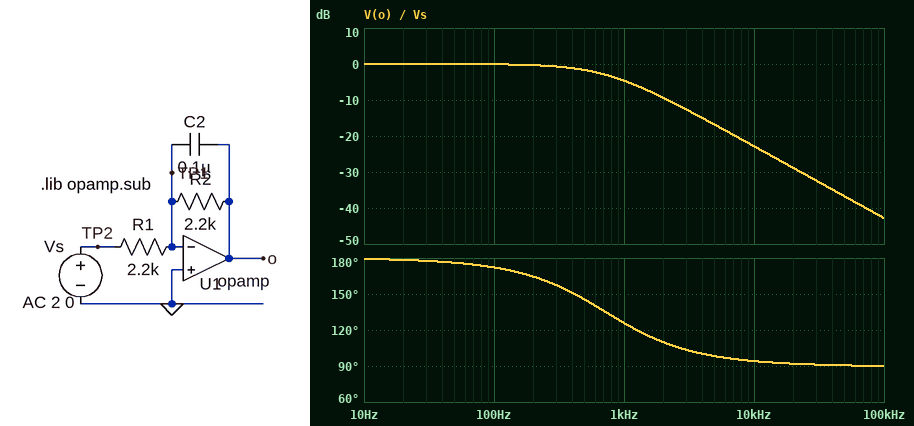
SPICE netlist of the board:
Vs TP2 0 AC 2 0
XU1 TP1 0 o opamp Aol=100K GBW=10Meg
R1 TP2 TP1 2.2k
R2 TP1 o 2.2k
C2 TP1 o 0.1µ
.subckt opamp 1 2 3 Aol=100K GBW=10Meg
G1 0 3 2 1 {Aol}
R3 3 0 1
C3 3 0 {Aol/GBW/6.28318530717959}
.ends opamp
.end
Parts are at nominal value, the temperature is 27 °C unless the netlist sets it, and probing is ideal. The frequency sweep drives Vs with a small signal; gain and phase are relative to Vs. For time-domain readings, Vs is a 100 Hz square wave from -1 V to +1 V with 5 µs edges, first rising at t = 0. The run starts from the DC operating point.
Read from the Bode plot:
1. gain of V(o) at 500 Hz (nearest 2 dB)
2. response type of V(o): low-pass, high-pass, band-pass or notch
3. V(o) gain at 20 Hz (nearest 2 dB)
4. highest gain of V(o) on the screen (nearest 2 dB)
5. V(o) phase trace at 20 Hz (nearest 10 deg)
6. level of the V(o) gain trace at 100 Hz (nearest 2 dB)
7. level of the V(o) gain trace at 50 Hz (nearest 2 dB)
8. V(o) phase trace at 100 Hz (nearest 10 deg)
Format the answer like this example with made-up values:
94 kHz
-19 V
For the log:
-2 dB
low-pass
0 dB
0 dB
180 deg
0 dB
0 dB
170 deg
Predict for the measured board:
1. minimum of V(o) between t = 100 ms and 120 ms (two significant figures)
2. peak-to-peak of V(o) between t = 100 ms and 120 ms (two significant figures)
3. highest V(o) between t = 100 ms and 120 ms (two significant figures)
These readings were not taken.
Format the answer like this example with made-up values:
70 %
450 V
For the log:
-1.0 V
2.0 V
1.0 V
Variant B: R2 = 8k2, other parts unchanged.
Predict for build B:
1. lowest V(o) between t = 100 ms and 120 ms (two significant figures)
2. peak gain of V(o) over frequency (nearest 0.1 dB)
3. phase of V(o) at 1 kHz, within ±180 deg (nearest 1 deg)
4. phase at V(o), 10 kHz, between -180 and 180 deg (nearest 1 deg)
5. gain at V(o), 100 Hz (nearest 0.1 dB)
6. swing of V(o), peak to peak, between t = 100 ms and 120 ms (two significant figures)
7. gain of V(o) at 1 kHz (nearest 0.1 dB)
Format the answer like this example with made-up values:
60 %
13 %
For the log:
-3.7 V
11.4 dB
101 deg
91 deg
10.4 dB
7.4 V
-3.0 dB
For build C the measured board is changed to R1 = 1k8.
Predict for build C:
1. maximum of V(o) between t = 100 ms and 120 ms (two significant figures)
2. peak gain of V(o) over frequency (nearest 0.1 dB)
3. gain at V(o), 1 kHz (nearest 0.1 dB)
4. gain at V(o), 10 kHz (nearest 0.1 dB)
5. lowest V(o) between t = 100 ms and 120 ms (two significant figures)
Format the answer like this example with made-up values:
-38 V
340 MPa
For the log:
1.2 V
1.7 dB
-2.9 dB
-21.1 dB
-1.2 V
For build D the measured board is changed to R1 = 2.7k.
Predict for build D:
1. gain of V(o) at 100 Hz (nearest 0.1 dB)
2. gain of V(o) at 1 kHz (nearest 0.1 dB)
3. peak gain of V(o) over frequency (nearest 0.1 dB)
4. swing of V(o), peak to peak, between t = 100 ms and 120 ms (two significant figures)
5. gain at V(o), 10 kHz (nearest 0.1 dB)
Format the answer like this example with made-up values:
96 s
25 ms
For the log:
-1.9 dB
-6.4 dB
-1.8 dB
1.6 V
-24.6 dB
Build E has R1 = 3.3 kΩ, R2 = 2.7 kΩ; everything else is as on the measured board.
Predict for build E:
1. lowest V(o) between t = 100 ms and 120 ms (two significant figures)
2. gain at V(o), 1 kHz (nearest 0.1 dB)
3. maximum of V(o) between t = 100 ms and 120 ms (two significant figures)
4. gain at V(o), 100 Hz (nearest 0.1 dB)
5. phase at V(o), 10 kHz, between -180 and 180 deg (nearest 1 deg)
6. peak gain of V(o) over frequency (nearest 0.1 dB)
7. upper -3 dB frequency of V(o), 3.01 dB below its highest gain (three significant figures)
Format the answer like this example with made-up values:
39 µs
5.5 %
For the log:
-820 mV
-7.6 dB
820 mV
-1.9 dB
93 deg
-1.7 dB
589 Hz
